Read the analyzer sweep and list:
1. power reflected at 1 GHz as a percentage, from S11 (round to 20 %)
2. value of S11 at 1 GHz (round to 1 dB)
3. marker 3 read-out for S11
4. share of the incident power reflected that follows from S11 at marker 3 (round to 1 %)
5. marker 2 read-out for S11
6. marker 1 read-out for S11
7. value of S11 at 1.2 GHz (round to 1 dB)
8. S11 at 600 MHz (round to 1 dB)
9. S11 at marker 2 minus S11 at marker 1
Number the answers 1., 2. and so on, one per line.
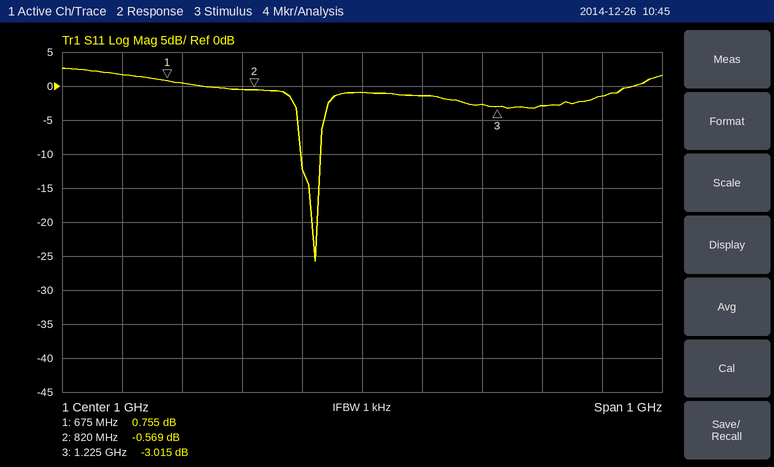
1. 80 %
2. -1 dB
3. -3.015 dB
4. 50 %
5. -0.569 dB
6. 0.755 dB
7. -3 dB
8. 2 dB
9. -1.324 dB
